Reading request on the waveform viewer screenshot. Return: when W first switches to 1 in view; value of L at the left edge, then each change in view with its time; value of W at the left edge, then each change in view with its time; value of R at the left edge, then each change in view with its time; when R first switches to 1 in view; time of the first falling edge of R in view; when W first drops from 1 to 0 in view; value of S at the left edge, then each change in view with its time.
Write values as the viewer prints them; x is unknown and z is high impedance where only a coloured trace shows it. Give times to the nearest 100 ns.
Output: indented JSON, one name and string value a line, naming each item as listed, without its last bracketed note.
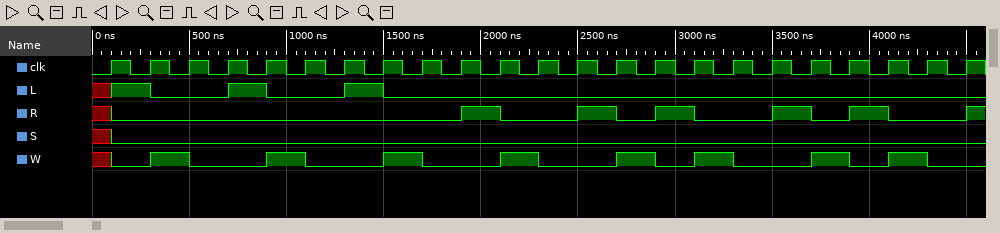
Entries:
{
  "when W first switches to 1 in view": "300 ns",
  "value of L at the left edge, then each change in view with its time": "x, 1 at 100 ns, 0 at 300 ns, 1 at 700 ns, 0 at 900 ns, 1 at 1300 ns, 0 at 1500 ns",
  "value of W at the left edge, then each change in view with its time": "x, 0 at 100 ns, 1 at 300 ns, 0 at 500 ns, 1 at 900 ns, 0 at 1100 ns, 1 at 1500 ns, 0 at 1700 ns, 1 at 2100 ns, 0 at 2300 ns, 1 at 2700 ns, 0 at 2900 ns, 1 at 3100 ns, 0 at 3300 ns, 1 at 3700 ns, 0 at 3900 ns, 1 at 4100 ns, 0 at 4300 ns",
  "value of R at the left edge, then each change in view with its time": "x, 0 at 100 ns, 1 at 1900 ns, 0 at 2100 ns, 1 at 2500 ns, 0 at 2700 ns, 1 at 2900 ns, 0 at 3100 ns, 1 at 3500 ns, 0 at 3700 ns, 1 at 3900 ns, 0 at 4100 ns, 1 at 4500 ns",
  "when R first switches to 1 in view": "1900 ns",
  "time of the first falling edge of R in view": "2100 ns",
  "when W first drops from 1 to 0 in view": "500 ns",
  "value of S at the left edge, then each change in view with its time": "x, 0 at 100 ns"
}
